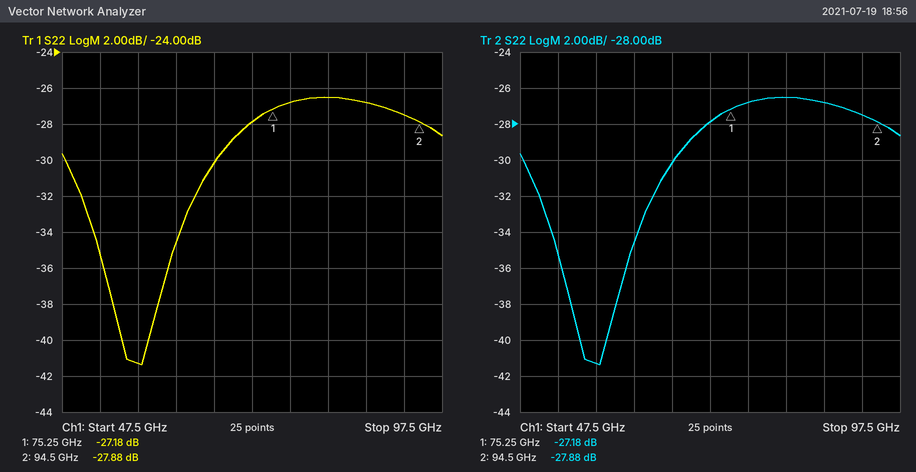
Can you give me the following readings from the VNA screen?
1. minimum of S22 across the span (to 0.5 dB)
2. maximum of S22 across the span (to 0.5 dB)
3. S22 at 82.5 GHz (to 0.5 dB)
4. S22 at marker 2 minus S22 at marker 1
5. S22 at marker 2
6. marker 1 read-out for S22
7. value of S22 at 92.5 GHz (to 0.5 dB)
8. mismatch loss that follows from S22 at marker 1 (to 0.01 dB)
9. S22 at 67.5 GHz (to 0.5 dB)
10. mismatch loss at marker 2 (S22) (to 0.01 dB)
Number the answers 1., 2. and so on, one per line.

1. -41.5 dB
2. -26.5 dB
3. -26.5 dB
4. -0.70 dB
5. -27.88 dB
6. -27.18 dB
7. -27.5 dB
8. 0.01 dB
9. -30.0 dB
10. 0.01 dB
